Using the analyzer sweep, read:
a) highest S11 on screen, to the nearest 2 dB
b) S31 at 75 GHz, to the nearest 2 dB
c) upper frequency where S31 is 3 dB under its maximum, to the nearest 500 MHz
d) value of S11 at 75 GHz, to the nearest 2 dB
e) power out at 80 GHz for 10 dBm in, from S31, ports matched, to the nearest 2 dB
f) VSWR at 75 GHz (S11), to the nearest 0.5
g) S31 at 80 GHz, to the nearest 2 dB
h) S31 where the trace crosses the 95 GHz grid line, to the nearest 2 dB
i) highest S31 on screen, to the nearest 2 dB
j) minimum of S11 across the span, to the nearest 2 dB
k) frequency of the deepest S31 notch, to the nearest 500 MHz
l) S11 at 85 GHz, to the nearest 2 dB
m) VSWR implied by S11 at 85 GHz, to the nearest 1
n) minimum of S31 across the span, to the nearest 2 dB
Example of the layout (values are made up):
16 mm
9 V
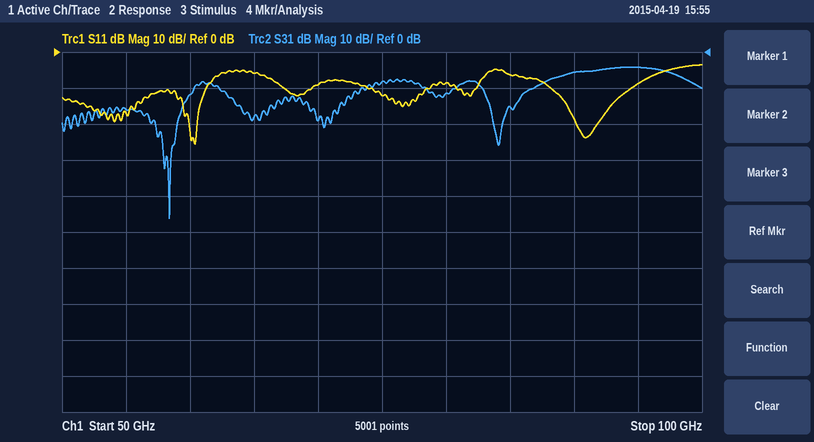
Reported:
-4 dB
-8 dB
98.5 GHz
-12 dB
-2 dBm
1.5
-12 dB
-4 dB
-4 dB
-26 dB
58.5 GHz
-6 dB
3
-46 dB
